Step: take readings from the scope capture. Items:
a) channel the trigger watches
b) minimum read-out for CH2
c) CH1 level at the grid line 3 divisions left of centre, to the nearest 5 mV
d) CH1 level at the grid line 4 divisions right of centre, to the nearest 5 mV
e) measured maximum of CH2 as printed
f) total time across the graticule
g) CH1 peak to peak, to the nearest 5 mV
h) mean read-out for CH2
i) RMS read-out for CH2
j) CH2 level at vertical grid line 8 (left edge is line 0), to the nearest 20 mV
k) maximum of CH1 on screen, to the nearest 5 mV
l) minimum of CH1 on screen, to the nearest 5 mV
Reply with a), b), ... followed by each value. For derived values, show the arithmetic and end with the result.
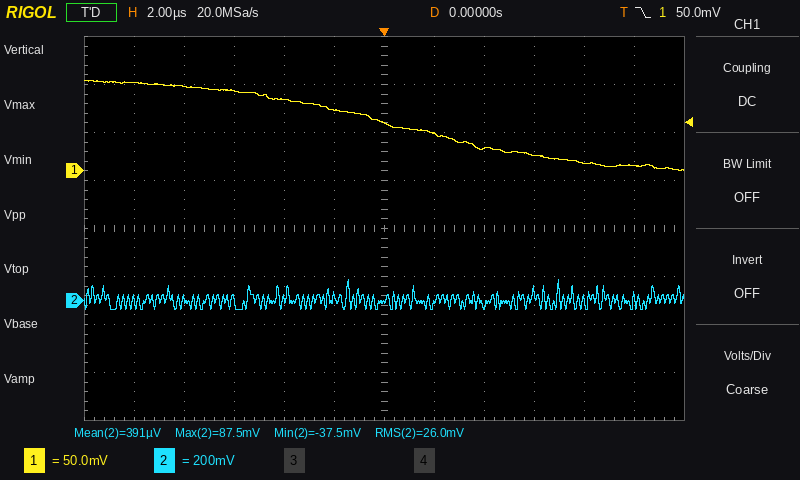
a) CH1
b) -37.5 mV
c) 85 mV
d) 10 mV
e) 87.5 mV
f) 24 µs
g) 95 mV − (0 mV) = 95 mV
h) 391 µV
i) 26.0 mV
j) -20 mV
k) 95 mV
l) 0 mV
